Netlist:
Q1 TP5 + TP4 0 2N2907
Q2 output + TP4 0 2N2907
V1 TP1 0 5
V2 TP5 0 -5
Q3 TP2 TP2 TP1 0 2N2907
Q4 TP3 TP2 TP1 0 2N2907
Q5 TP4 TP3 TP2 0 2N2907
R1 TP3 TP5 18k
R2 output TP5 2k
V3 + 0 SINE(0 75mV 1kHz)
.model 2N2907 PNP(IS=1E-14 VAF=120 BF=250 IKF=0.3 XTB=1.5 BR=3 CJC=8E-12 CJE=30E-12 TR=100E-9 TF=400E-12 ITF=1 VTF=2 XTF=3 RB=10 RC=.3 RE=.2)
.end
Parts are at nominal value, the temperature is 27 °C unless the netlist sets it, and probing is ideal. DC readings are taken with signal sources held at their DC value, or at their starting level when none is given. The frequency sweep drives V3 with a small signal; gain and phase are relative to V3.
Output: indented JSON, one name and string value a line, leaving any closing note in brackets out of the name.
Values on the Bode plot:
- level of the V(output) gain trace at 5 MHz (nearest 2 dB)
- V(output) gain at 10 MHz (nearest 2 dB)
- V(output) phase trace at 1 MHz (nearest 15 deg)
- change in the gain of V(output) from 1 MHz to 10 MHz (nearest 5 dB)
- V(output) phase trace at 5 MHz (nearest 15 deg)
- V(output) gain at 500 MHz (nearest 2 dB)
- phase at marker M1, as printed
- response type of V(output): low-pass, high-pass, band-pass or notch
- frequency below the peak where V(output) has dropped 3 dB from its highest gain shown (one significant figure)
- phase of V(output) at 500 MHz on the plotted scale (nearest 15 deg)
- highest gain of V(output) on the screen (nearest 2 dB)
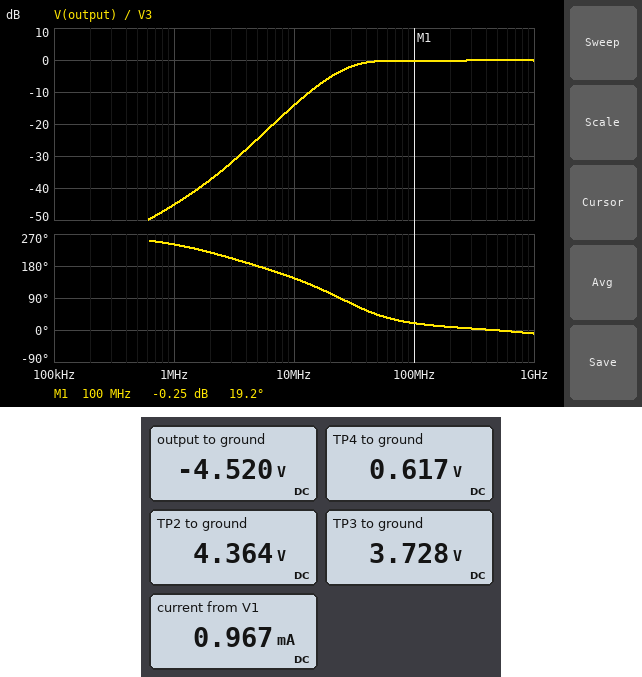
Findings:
{
  "level of the V(output) gain trace at 5 MHz": "-24 dB",
  "V(output) gain at 10 MHz": "-14 dB",
  "V(output) phase trace at 1 MHz": "240 deg",
  "change in the gain of V(output) from 1 MHz to 10 MHz": "30 dB",
  "V(output) phase trace at 5 MHz": "180 deg",
  "V(output) gain at 500 MHz": "0 dB",
  "phase at marker M1, as printed": "19.2 deg",
  "response type of V(output): low-pass, high-pass, band-pass or notch": "high-pass",
  "frequency below the peak where V(output) has dropped 3 dB from its highest gain shown": "30 MHz",
  "phase of V(output) at 500 MHz on the plotted scale": "0 deg",
  "highest gain of V(output) on the screen": "0 dB"
}
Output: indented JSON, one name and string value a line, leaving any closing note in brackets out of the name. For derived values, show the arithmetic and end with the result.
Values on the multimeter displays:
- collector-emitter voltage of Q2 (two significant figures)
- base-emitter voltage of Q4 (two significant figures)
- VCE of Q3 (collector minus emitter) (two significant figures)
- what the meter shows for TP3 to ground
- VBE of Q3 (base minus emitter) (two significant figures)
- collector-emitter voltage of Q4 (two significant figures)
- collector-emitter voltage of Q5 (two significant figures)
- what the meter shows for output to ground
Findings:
{
  "collector-emitter voltage of Q2": "-4.52 V - 617 mV = -5.1 V",
  "base-emitter voltage of Q4": "4.364 V - 5 V = -640 mV",
  "VCE of Q3 (collector minus emitter)": "4.364 V - 5 V = -640 mV",
  "what the meter shows for TP3 to ground": "3.728 V",
  "VBE of Q3 (base minus emitter)": "4.364 V - 5 V = -640 mV",
  "collector-emitter voltage of Q4": "3.728 V - 5 V = -1.3 V",
  "collector-emitter voltage of Q5": "617 mV - 4.364 V = -3.7 V",
  "what the meter shows for output to ground": "-4.520 V"
}
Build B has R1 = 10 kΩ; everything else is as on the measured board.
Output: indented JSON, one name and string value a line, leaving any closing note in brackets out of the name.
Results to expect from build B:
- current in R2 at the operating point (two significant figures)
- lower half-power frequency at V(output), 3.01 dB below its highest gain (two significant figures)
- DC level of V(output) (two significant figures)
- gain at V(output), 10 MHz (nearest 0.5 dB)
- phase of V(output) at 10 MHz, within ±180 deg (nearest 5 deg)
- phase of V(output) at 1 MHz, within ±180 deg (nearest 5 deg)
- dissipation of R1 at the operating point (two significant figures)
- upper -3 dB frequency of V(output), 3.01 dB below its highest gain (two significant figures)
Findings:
{
  "current in R2 at the operating point": "430 µA",
  "lower half-power frequency at V(output), 3.01 dB below its highest gain": "38 MHz",
  "DC level of V(output)": "-4.1 V",
  "gain at V(output), 10 MHz": "-18.5 dB",
  "phase of V(output) at 10 MHz, within ±180 deg": "155 deg",
  "phase of V(output) at 1 MHz, within ±180 deg": "-115 deg",
  "dissipation of R1 at the operating point": "7.6 mW",
  "upper -3 dB frequency of V(output), 3.01 dB below its highest gain": "4.2 GHz"
}
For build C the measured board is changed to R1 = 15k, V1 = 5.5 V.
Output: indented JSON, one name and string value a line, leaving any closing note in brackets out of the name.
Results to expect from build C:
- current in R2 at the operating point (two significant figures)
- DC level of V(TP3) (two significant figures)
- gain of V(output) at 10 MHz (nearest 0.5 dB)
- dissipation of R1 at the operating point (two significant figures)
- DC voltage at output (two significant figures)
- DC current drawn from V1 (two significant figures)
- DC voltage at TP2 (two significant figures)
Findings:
{
  "current in R2 at the operating point": "300 µA",
  "DC level of V(TP3)": "4.2 V",
  "gain of V(output) at 10 MHz": "-16.0 dB",
  "dissipation of R1 at the operating point": "5.7 mW",
  "DC voltage at output": "-4.4 V",
  "DC current drawn from V1": "1.2 mA",
  "DC voltage at TP2": "4.9 V"
}
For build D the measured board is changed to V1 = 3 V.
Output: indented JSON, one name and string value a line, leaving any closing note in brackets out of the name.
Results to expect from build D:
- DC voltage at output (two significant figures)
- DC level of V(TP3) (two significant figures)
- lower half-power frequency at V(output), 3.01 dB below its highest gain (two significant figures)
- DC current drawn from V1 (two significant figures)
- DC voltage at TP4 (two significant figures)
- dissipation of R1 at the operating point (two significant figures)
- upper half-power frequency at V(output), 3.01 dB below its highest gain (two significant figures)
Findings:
{
  "DC voltage at output": "-4.6 V",
  "DC level of V(TP3)": "1.7 V",
  "lower half-power frequency at V(output), 3.01 dB below its highest gain": "20 MHz",
  "DC current drawn from V1": "750 µA",
  "DC voltage at TP4": "610 mV",
  "dissipation of R1 at the operating point": "2.5 mW",
  "upper half-power frequency at V(output), 3.01 dB below its highest gain": "3.8 GHz"
}
